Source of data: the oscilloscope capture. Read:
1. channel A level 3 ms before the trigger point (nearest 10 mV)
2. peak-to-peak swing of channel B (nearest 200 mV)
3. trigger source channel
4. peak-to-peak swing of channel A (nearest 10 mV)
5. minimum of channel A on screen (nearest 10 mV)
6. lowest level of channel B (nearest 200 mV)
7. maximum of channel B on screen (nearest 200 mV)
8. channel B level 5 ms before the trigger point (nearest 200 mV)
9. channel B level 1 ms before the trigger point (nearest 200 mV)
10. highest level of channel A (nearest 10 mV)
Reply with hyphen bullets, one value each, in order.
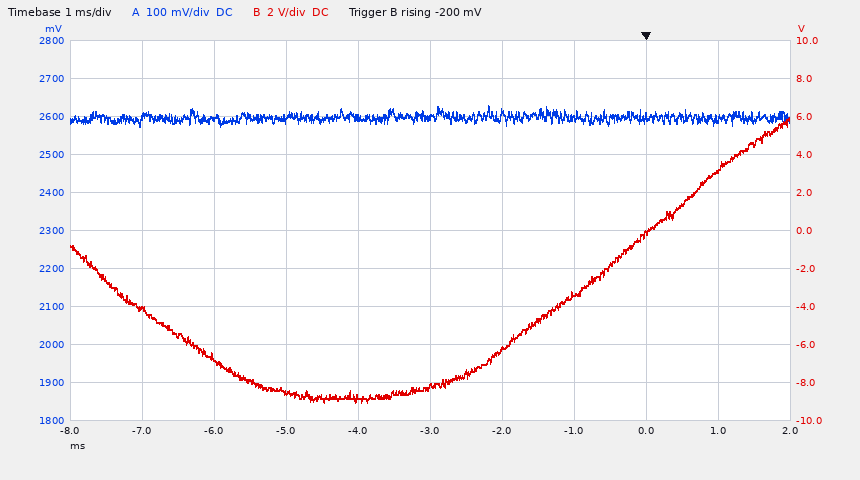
- 2.60 V
- 15.0 V
- channel B
- 60 mV
- 2.57 V
- -9.0 V
- 6.0 V
- -8.6 V
- -3.4 V
- 2.63 V
